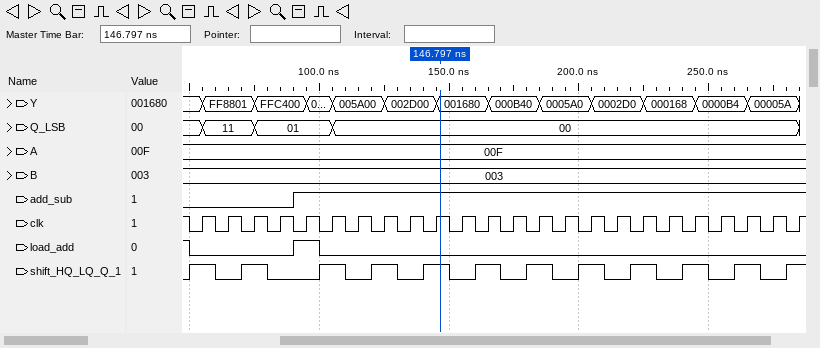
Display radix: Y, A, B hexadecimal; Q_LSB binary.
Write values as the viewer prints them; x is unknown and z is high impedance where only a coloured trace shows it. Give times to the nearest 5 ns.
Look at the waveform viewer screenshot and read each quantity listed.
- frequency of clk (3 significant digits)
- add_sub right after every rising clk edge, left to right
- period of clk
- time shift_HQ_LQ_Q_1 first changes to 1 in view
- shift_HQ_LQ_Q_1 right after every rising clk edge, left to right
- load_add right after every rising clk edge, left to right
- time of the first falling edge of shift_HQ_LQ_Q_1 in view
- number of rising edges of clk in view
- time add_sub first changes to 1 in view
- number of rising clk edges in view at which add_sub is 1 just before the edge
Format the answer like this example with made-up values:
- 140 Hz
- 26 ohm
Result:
- 100 MHz
- 0 0 0 0 1 1 1 1 1 1 1 1 1 1 1 1 1 1 1 1 1 1 1 1
- 10 ns
- 50 ns
- 1 0 1 0 0 1 0 1 0 1 0 1 0 1 0 1 0 1 0 1 0 1 0 1
- 0 0 0 0 1 0 0 0 0 0 0 0 0 0 0 0 0 0 0 0 0 0 0 0
- 60 ns
- 24
- 90 ns
- 20
